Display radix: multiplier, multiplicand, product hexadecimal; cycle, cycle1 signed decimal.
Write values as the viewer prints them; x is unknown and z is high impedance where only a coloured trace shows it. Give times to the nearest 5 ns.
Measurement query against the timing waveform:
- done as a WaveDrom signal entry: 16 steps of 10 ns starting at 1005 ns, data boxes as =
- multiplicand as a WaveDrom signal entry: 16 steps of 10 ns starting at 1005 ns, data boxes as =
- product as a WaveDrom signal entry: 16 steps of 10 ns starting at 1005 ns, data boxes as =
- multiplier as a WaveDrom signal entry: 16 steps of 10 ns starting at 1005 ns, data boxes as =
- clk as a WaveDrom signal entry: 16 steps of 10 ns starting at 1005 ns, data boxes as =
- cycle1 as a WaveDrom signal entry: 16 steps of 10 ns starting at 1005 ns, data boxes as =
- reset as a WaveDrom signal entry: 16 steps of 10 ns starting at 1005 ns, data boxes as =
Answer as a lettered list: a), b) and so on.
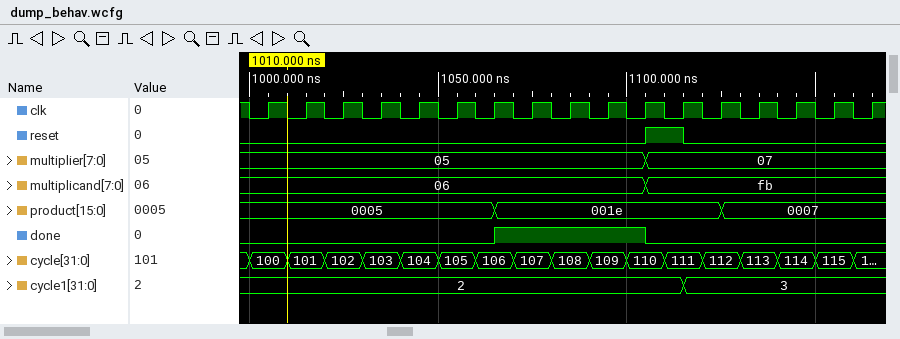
a) {name: 'done', wave: '0.....1...0.....'}
b) {name: 'multiplicand', wave: '=.........=.....', data: '06 fb'}
c) {name: 'product', wave: '=.....=.....=...', data: '0005 001e 0007'}
d) {name: 'multiplier', wave: '=.........=.....', data: '05 07'}
e) {name: 'clk', wave: 'p...............'}
f) {name: 'cycle1', wave: '=..........=....', data: '2 3'}
g) {name: 'reset', wave: '0.........10....'}
